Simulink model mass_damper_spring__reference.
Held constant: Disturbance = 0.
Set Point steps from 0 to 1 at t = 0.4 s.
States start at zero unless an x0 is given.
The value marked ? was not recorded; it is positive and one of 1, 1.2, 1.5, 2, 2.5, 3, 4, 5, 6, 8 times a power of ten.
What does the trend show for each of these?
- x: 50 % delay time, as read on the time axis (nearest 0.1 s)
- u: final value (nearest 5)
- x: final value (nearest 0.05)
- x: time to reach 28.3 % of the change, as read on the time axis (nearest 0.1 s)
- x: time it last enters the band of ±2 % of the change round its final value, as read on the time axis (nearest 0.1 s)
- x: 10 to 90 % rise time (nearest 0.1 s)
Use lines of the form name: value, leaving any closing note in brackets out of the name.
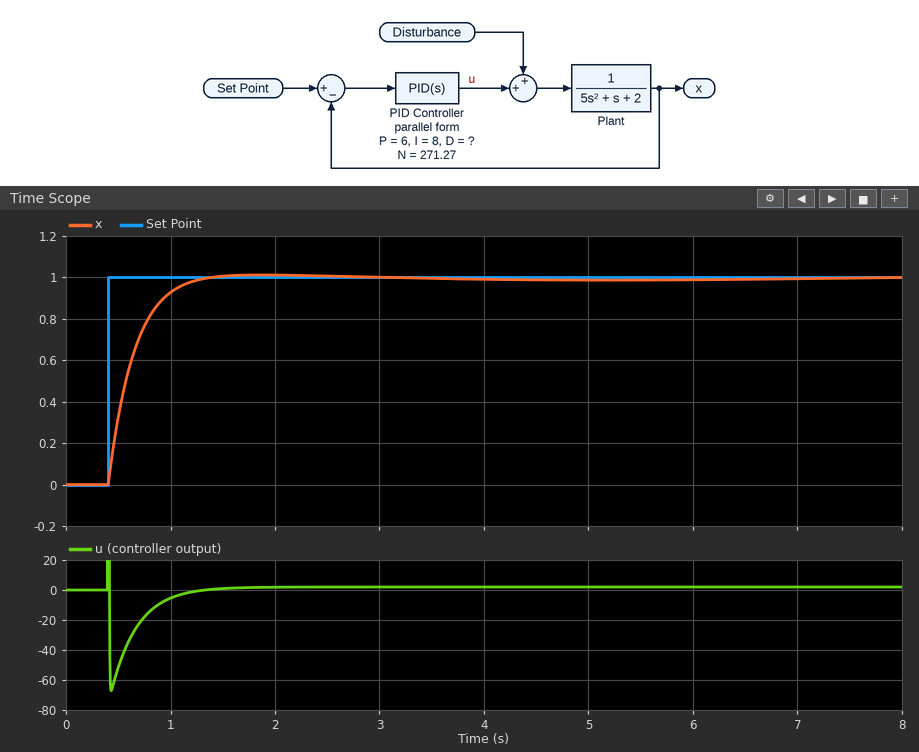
x: 50 % delay time, as read on the time axis: 0.6 s
u: final value: 0
x: final value: 1.00
x: time to reach 28.3 % of the change, as read on the time axis: 0.5 s
x: time it last enters the band of ±2 % of the change round its final value, as read on the time axis: 1.2 s
x: 10 to 90 % rise time: 0.5 s
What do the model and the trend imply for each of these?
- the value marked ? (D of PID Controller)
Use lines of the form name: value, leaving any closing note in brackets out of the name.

the value marked ?: 20
